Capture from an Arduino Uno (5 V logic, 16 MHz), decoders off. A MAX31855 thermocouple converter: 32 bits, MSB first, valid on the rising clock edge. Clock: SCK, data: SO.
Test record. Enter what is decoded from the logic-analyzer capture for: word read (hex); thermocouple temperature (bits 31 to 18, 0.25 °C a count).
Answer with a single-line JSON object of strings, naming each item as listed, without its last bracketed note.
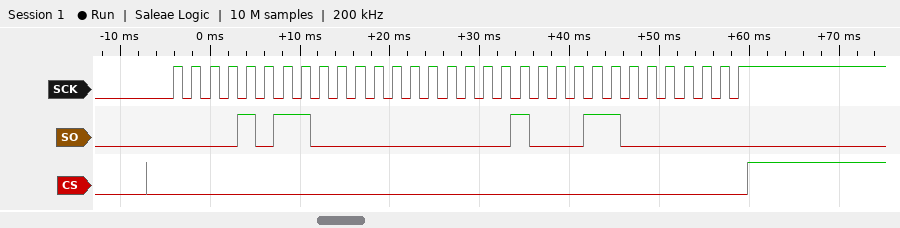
{"word read": "0x0B001180", "thermocouple temperature": "176.00 °C"}
